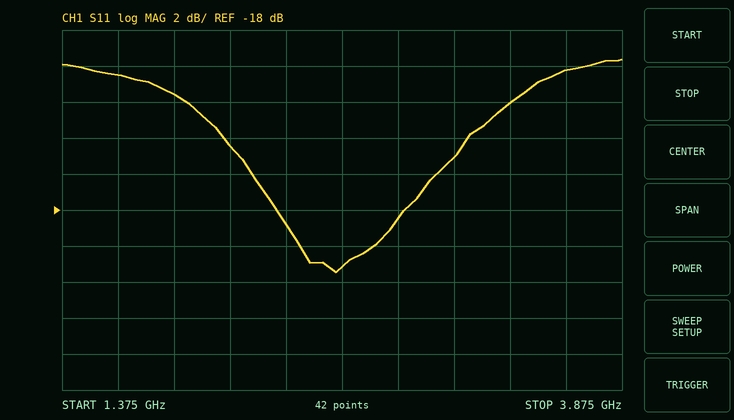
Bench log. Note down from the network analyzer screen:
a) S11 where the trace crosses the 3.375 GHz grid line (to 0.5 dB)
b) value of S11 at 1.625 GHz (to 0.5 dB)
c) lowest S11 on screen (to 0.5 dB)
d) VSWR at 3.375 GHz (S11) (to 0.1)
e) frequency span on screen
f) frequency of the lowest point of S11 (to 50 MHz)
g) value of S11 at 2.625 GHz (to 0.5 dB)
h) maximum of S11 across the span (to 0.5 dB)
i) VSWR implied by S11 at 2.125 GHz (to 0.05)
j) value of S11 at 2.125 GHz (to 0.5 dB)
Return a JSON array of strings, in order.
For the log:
["-12.0 dB", "-10.5 dB", "-21.5 dB", "1.7", "2.5 GHz", "2.60 GHz", "-21.0 dB", "-9.5 dB", "1.45", "-14.5 dB"]
